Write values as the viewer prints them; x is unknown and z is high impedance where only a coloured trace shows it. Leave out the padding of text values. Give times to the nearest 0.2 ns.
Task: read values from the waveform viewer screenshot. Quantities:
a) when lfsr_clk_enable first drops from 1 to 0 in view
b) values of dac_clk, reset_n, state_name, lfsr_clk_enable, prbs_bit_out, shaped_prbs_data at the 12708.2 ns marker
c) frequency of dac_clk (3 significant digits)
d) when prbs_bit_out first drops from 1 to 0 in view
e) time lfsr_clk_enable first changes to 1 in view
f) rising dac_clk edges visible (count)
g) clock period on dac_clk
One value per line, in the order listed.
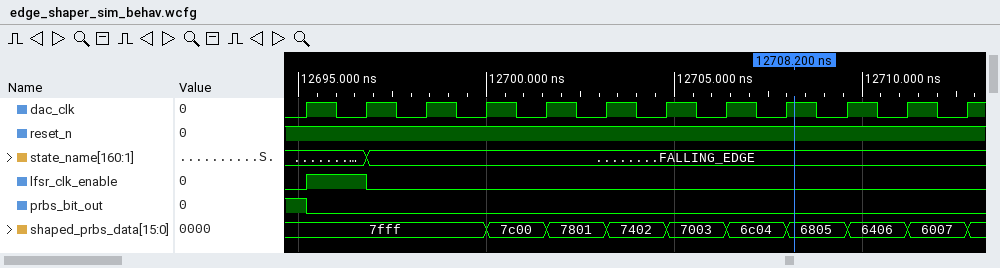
12696.8 ns
dac_clk=1, reset_n=1, state_name=FALLING_EDGE, lfsr_clk_enable=0, prbs_bit_out=0, shaped_prbs_data=6805
625 MHz
12695.2 ns
12695.2 ns
12
1.6 ns
